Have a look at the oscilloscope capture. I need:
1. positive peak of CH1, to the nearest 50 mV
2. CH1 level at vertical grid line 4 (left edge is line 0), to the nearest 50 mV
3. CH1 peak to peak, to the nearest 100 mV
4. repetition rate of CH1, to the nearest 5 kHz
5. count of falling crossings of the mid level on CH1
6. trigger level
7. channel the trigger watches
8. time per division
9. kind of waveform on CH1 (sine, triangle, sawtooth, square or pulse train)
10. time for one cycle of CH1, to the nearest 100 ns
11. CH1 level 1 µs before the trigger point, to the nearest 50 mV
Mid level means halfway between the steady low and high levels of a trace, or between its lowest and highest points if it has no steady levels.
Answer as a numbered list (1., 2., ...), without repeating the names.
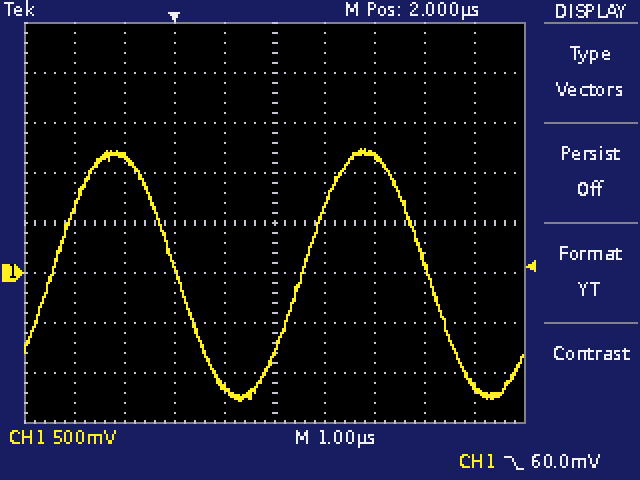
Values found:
1. 1.25 V
2. -1.15 V
3. 2.50 V
4. 200 kHz
5. 2
6. 60.0 mV
7. CH1
8. 1 µs
9. sine
10. 5.0 µs
11. 1.15 V
